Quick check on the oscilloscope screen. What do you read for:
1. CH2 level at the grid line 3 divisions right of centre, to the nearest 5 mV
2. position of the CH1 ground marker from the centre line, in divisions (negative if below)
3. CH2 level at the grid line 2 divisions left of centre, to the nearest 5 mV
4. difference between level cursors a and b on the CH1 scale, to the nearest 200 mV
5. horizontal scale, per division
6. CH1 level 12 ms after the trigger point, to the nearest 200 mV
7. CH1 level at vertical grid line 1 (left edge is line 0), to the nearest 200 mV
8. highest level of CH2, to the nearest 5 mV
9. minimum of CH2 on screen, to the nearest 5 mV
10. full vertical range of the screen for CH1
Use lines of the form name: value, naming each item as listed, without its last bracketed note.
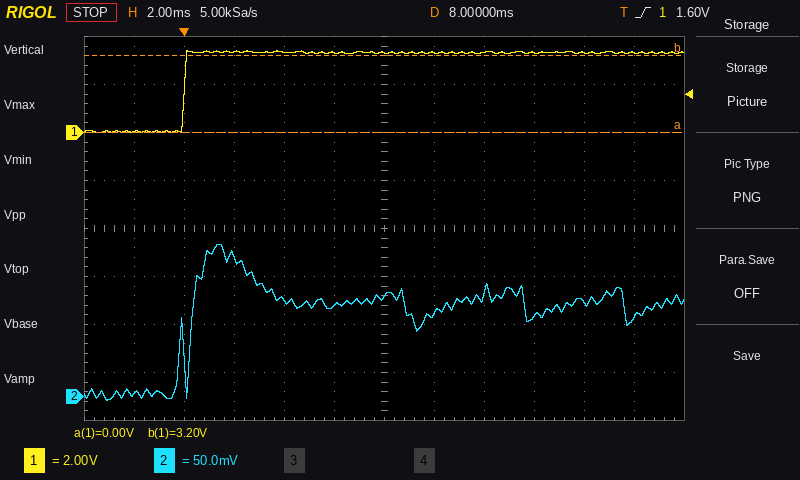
CH2 level at the grid line 3 divisions right of centre, to the nearest 5 mV: 85 mV
position of the CH1 ground marker from the centre line, in divisions: +2.0 div
CH2 level at the grid line 2 divisions left of centre, to the nearest 5 mV: 100 mV
difference between level cursors a and b on the CH1 scale, to the nearest 200 mV: 3.2 V
horizontal scale, per division: 2 ms
CH1 level 12 ms after the trigger point, to the nearest 200 mV: 3.4 V
CH1 level at vertical grid line 1 (left edge is line 0), to the nearest 200 mV: 0.0 V
highest level of CH2, to the nearest 5 mV: 160 mV
minimum of CH2 on screen, to the nearest 5 mV: -5 mV
full vertical range of the screen for CH1: 16 V
